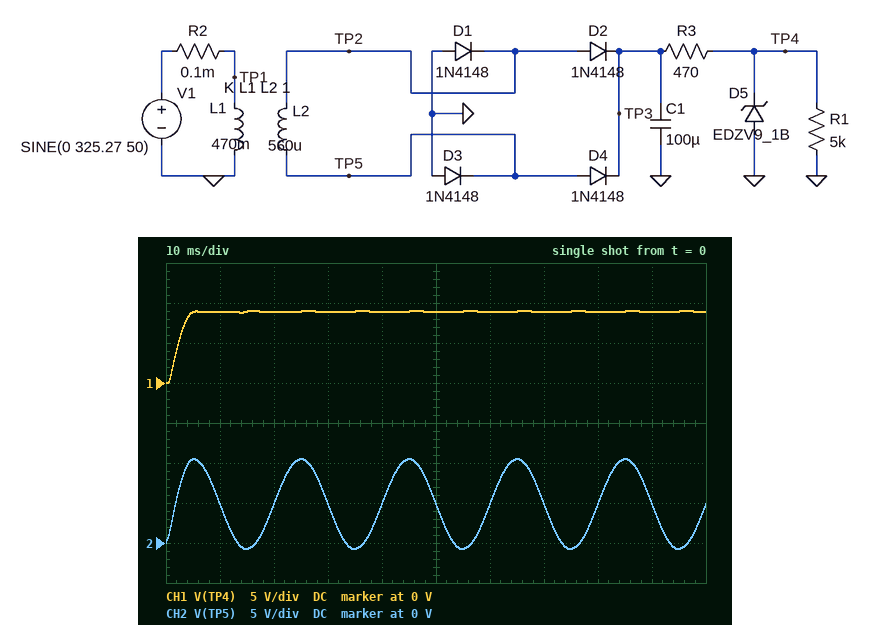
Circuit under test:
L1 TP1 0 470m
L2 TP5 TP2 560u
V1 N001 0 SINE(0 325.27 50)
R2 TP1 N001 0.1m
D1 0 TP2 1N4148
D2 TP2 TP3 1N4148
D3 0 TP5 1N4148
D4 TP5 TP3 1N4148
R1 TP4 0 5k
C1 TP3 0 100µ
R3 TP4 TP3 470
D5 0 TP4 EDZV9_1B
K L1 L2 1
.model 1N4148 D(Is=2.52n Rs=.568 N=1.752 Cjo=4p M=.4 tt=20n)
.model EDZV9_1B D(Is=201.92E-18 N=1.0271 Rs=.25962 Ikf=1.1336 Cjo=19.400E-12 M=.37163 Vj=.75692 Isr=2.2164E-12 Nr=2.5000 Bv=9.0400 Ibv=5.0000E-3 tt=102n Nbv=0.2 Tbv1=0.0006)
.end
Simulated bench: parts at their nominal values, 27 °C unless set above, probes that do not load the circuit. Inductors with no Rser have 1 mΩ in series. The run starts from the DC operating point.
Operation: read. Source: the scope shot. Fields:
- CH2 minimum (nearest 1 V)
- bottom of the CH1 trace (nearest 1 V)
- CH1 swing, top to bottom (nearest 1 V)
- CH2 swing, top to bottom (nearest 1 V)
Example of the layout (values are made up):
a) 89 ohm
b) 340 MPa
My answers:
a) -1 V
b) 0 V
c) 9 V
d) 11 V
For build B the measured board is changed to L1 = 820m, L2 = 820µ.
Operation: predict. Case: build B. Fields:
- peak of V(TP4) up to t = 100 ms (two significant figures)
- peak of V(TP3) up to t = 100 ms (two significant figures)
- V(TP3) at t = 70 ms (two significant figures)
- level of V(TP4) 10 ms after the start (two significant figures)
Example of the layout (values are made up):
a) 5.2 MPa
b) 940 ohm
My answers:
a) 8.1 V
b) 8.9 V
c) 8.8 V
d) 8.0 V
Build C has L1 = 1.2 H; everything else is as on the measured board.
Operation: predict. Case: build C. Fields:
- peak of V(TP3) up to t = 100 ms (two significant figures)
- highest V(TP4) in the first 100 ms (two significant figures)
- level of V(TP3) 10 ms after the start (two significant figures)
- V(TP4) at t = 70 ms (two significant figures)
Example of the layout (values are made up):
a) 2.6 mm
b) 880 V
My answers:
a) 5.7 V
b) 5.2 V
c) 5.6 V
d) 5.1 V
